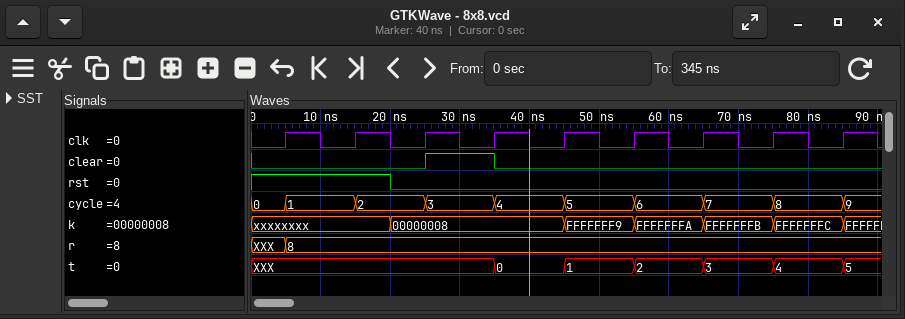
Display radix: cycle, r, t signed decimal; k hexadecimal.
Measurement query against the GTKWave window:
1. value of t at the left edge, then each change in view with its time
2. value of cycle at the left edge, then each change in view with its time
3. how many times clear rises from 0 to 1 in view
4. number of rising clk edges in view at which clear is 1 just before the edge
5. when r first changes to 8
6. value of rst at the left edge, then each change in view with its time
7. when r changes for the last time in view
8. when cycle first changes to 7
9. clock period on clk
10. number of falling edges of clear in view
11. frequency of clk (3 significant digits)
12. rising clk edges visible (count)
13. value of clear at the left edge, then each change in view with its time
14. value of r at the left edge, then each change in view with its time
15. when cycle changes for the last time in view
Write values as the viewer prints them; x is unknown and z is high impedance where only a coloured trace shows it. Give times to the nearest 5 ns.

XXX, 0 at 35 ns, 1 at 45 ns, 2 at 55 ns, 3 at 65 ns, 4 at 75 ns, 5 at 85 ns
0, 1 at 5 ns, 2 at 15 ns, 3 at 25 ns, 4 at 35 ns, 5 at 45 ns, 6 at 55 ns, 7 at 65 ns, 8 at 75 ns, 9 at 85 ns
1
1
5 ns
1, 0 at 20 ns
5 ns
65 ns
10 ns
1
100 MHz
9
0, 1 at 25 ns, 0 at 35 ns
XXX, 8 at 5 ns
85 ns
